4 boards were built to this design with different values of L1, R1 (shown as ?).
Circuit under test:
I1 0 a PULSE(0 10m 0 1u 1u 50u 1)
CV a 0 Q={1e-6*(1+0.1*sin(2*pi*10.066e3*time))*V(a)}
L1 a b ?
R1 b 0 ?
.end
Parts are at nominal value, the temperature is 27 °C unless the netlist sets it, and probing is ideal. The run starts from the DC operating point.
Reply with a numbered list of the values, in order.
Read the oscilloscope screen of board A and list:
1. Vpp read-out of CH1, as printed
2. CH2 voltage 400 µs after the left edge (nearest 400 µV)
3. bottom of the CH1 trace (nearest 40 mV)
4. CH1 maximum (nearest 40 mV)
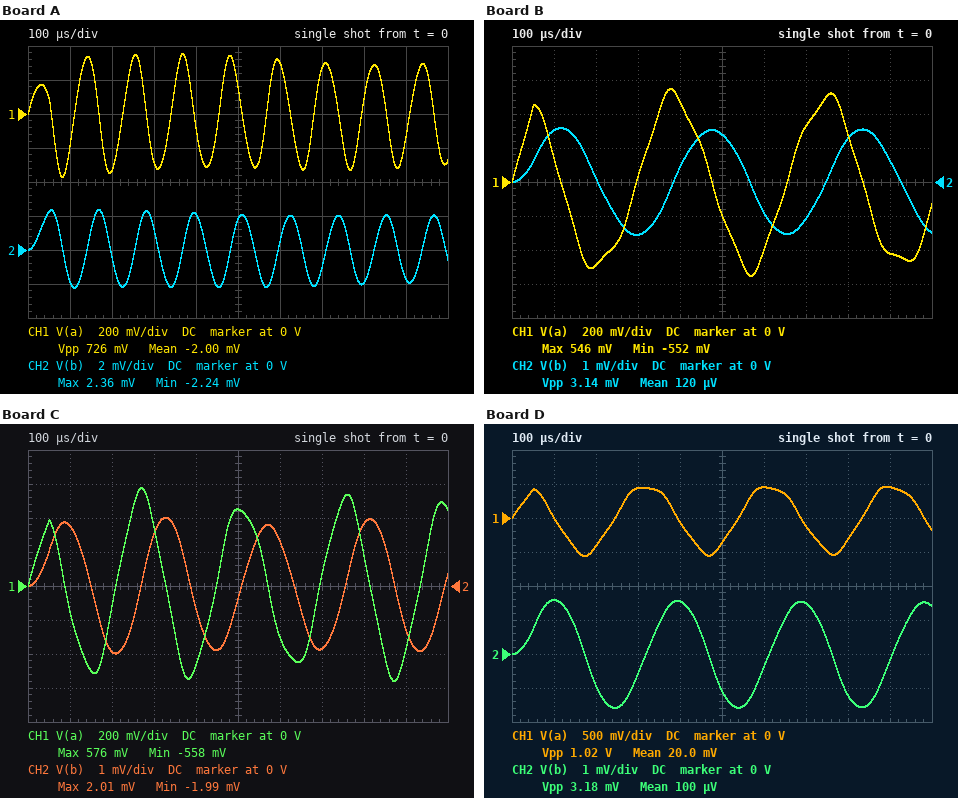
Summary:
1. 726 mV
2. 2.0 mV
3. -360 mV
4. 360 mV
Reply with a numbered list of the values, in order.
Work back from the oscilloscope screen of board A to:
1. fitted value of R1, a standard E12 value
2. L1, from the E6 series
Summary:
1. 0.12 Ω
2. 330 µH
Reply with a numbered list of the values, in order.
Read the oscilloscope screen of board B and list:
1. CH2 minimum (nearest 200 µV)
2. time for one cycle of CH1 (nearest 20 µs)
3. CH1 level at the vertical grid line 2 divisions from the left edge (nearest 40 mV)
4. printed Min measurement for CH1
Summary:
1. -1.6 mV
2. 360 µs
3. -480 mV
4. -552 mV
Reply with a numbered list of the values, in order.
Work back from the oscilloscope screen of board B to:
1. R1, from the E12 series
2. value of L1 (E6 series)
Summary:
1. 0.18 Ω
2. 3.3 mH
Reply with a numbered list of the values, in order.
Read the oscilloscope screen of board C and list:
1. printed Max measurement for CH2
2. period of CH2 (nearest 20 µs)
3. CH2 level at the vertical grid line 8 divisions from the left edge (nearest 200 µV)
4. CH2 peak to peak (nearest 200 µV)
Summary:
1. 2.01 mV
2. 240 µs
3. 1.8 mV
4. 4.0 mV
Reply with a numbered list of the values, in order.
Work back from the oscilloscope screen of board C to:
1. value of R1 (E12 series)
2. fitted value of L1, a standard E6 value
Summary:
1. 0.15 Ω
2. 1.5 mH
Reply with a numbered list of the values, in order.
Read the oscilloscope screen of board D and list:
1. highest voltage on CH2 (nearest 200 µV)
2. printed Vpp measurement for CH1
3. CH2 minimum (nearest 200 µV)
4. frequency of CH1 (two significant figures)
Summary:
1. 1.6 mV
2. 1.02 V
3. -1.6 mV
4. 3.4 kHz
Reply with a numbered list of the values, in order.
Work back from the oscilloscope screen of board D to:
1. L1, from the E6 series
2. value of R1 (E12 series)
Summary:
1. 2.2 mH
2. 0.15 Ω
